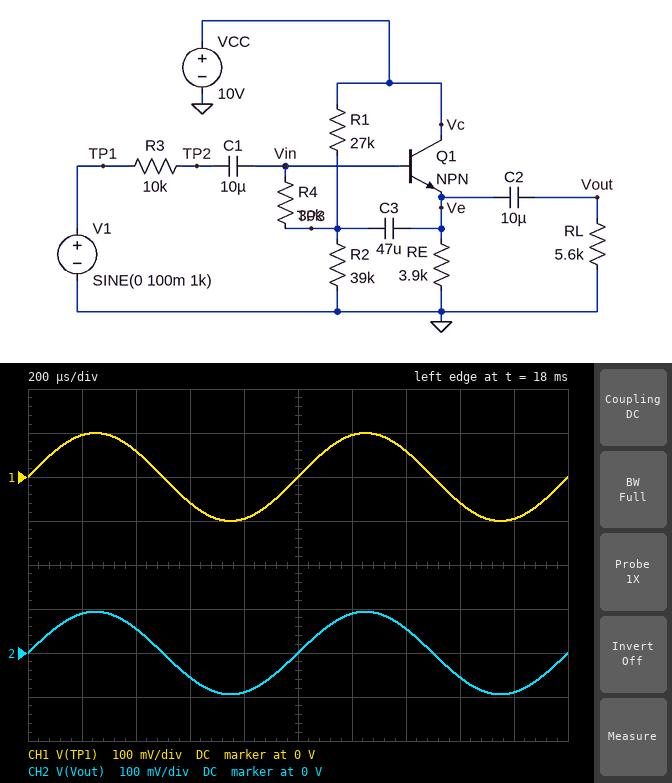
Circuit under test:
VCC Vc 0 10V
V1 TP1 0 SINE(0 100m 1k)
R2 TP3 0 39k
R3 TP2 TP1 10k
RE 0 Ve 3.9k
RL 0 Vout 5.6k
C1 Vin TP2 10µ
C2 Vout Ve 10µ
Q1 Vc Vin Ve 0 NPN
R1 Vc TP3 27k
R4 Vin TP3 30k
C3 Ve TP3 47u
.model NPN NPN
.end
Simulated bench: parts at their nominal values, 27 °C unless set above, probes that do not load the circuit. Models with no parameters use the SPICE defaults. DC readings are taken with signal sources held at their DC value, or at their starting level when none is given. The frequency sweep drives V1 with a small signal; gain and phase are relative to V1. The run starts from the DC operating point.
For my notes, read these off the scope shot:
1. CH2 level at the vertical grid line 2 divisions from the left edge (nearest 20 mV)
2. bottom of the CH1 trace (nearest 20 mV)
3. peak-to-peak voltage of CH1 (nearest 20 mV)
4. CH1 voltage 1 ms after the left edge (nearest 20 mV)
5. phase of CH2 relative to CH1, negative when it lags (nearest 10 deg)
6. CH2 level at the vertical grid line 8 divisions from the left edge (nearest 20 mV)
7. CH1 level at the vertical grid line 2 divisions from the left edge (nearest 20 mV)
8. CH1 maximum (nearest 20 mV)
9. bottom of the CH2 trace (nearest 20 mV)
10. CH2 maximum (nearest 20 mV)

60 mV
-100 mV
200 mV
0 V
0 deg
-60 mV
60 mV
100 mV
-100 mV
100 mV
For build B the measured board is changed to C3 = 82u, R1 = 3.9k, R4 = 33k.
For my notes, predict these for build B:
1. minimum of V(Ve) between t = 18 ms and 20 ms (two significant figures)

7.5 V
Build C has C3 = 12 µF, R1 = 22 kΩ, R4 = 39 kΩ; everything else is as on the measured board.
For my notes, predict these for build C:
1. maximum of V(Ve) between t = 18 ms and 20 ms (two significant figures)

5.0 V
